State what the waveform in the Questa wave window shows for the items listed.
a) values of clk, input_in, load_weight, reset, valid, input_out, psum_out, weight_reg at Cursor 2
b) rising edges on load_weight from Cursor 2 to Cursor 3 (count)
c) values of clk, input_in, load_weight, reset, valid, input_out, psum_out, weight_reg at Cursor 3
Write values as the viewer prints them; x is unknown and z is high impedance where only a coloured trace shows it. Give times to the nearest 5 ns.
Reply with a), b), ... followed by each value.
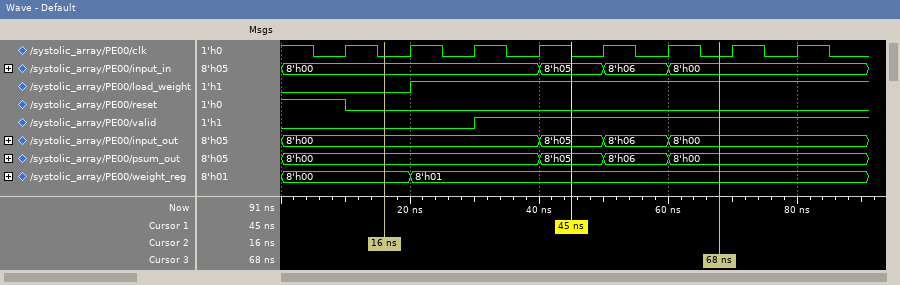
a) clk=0, input_in=8'h00, load_weight=0, reset=0, valid=0, input_out=8'h00, psum_out=8'h00, weight_reg=8'h00
b) 1
c) clk=0, input_in=8'h00, load_weight=1, reset=0, valid=1, input_out=8'h00, psum_out=8'h00, weight_reg=8'h01
